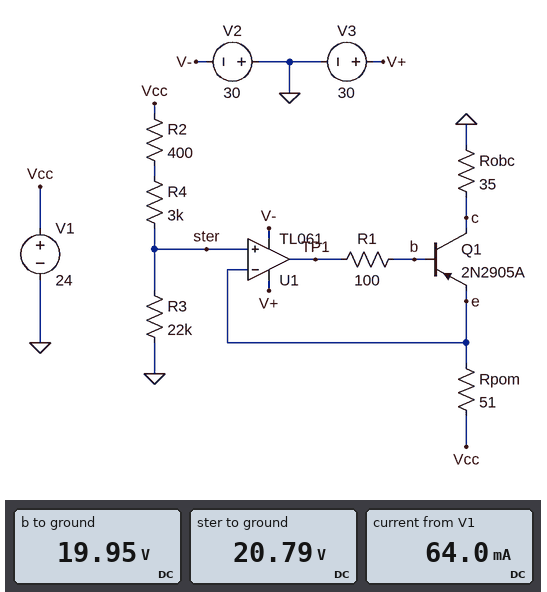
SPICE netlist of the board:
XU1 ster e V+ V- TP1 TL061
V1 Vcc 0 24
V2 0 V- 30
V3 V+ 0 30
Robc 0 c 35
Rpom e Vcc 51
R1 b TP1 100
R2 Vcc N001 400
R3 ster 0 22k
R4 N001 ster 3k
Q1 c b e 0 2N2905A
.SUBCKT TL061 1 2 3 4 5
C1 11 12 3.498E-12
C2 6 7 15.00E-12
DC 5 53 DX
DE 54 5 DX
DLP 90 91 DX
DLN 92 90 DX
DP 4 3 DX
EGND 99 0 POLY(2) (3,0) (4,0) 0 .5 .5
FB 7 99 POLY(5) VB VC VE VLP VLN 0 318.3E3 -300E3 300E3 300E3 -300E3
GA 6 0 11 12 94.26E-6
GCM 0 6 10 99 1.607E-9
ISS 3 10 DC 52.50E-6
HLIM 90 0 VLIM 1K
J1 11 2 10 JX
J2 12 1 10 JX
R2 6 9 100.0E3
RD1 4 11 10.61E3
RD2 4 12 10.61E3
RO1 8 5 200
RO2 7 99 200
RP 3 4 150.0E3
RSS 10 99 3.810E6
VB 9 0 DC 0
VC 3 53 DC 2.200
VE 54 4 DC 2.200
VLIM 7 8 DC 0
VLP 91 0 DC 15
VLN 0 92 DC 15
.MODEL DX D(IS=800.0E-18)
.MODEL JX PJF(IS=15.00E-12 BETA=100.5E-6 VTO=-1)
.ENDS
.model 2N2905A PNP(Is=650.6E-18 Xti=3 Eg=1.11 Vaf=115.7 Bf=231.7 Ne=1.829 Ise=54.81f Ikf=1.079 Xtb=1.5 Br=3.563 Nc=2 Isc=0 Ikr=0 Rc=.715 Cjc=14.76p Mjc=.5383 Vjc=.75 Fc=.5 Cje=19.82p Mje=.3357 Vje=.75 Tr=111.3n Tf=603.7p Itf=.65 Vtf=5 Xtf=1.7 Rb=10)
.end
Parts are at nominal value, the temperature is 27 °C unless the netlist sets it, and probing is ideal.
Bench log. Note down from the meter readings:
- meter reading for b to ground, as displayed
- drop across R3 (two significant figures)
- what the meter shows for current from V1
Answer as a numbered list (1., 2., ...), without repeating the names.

1. 19.95 V
2. 21 V
3. 64.0 mA
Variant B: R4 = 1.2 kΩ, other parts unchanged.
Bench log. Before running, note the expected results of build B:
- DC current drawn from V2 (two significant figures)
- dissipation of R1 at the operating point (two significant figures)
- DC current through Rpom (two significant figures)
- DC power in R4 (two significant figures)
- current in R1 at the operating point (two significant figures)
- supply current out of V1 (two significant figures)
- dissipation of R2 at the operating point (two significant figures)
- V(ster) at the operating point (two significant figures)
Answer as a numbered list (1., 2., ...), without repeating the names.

1. 450 µA
2. 1.5 µW
3. 32 mA
4. 1.2 mW
5. 120 µA
6. 33 mA
7. 410 µW
8. 22 V
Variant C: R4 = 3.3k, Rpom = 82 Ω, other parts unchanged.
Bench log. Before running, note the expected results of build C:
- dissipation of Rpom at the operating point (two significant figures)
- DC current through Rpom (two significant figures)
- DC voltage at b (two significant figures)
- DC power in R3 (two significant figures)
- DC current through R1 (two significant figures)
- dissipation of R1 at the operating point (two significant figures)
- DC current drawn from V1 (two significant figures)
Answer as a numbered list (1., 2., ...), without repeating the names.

1. 150 mW
2. 42 mA
3. 20 V
4. 19 mW
5. 160 µA
6. 2.7 µW
7. 43 mA
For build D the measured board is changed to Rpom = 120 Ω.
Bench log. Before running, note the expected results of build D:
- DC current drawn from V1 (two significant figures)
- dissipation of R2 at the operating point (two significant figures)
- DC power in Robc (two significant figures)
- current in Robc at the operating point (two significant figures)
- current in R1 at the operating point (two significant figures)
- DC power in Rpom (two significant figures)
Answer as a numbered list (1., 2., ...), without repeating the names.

1. 28 mA
2. 360 µW
3. 25 mW
4. 27 mA
5. 100 µA
6. 86 mW
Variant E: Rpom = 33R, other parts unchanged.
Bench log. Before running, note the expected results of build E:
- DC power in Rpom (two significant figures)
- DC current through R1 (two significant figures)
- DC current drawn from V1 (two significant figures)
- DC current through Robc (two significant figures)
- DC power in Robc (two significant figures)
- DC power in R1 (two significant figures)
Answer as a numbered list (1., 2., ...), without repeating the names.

1. 310 mW
2. 400 µA
3. 98 mA
4. 97 mA
5. 330 mW
6. 16 µW
